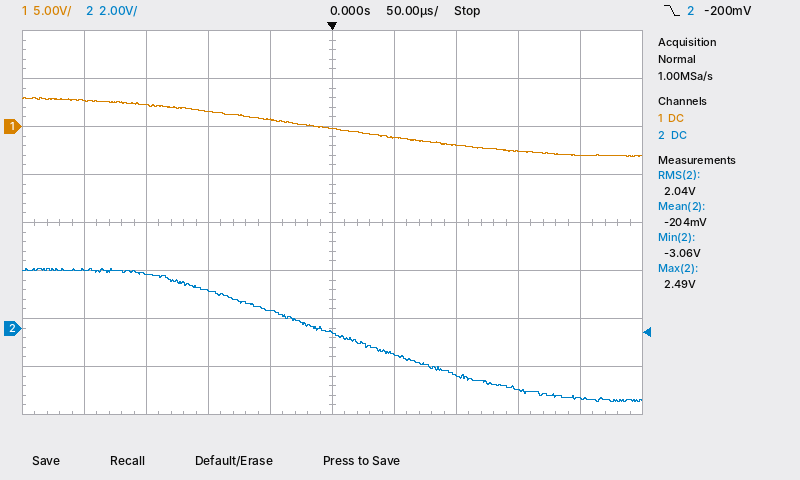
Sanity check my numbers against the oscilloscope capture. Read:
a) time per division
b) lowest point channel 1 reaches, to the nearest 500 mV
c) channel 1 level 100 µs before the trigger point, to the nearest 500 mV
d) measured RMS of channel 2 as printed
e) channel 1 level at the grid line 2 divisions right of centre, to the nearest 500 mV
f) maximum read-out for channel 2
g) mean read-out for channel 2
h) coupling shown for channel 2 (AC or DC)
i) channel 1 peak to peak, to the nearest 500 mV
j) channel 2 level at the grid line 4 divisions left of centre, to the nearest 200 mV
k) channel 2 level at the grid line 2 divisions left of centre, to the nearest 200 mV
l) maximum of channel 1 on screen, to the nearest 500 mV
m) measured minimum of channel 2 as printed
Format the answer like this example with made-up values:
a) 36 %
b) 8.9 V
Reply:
a) 50 µs
b) -3.0 V
c) 1.5 V
d) 2.04 V
e) -2.0 V
f) 2.49 V
g) -204 mV
h) DC
i) 6.0 V
j) 2.4 V
k) 1.6 V
l) 3.0 V
m) -3.06 V
